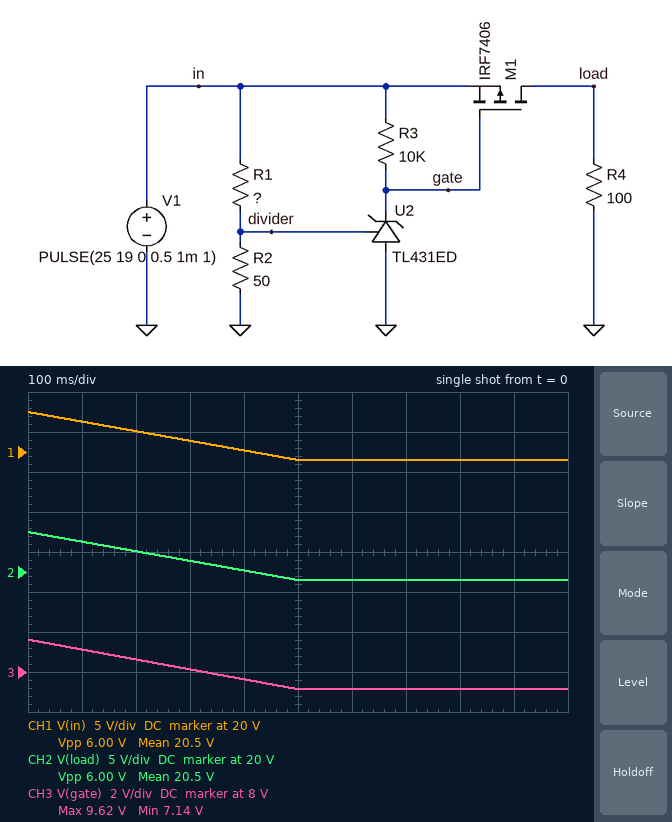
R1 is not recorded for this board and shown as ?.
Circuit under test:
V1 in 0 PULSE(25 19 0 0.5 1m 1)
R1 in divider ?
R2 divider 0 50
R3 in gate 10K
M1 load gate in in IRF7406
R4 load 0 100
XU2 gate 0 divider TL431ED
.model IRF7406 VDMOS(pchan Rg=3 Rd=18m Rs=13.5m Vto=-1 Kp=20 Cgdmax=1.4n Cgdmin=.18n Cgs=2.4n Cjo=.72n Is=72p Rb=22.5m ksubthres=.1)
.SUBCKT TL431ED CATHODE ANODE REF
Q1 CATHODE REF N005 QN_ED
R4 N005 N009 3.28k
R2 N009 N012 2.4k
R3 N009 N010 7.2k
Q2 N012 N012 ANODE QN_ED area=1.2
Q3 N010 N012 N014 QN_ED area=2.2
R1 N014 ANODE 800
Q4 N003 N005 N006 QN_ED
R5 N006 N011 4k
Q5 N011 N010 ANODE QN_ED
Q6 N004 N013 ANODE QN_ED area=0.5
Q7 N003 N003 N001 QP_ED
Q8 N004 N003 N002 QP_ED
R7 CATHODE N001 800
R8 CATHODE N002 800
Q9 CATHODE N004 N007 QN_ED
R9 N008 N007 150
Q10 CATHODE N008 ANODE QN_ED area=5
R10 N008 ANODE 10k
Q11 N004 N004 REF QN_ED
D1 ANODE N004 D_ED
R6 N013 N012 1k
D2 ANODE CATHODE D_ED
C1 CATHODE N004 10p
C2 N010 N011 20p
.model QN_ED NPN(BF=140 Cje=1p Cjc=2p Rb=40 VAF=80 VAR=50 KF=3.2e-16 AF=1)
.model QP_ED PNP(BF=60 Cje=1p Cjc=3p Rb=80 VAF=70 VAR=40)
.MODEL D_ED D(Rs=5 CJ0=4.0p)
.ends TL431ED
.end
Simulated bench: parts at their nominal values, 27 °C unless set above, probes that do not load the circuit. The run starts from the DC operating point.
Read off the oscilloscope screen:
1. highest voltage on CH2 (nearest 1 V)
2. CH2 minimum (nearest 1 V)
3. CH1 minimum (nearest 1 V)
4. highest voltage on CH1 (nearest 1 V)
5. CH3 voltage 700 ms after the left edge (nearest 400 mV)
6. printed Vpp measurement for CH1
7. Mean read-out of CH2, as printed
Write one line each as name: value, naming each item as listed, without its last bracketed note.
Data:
highest voltage on CH2: 25 V
CH2 minimum: 19 V
CH1 minimum: 19 V
highest voltage on CH1: 25 V
CH3 voltage 700 ms after the left edge: 7.2 V
printed Vpp measurement for CH1: 6.00 V
Mean read-out of CH2, as printed: 20.5 V
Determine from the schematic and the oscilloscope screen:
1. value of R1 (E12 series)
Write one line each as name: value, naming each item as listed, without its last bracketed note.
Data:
value of R1: 68 Ω
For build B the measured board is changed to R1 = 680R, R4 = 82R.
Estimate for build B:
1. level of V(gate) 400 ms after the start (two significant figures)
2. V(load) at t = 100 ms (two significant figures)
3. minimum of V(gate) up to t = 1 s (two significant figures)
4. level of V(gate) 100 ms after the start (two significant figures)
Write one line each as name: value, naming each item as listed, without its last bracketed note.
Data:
level of V(gate) 400 ms after the start: 20 V
V(load) at t = 100 ms: 1.4 mV
minimum of V(gate) up to t = 1 s: 19 V
level of V(gate) 100 ms after the start: 23 V
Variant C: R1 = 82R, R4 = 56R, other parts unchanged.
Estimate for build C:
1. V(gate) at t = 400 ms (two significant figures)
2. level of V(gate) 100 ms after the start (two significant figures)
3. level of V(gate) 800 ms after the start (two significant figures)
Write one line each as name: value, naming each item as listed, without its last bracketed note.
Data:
V(gate) at t = 400 ms: 6.8 V
level of V(gate) 100 ms after the start: 8.1 V
level of V(gate) 800 ms after the start: 6.3 V
